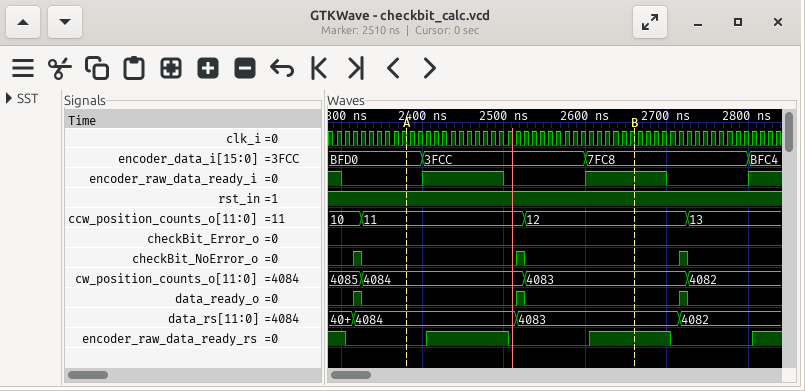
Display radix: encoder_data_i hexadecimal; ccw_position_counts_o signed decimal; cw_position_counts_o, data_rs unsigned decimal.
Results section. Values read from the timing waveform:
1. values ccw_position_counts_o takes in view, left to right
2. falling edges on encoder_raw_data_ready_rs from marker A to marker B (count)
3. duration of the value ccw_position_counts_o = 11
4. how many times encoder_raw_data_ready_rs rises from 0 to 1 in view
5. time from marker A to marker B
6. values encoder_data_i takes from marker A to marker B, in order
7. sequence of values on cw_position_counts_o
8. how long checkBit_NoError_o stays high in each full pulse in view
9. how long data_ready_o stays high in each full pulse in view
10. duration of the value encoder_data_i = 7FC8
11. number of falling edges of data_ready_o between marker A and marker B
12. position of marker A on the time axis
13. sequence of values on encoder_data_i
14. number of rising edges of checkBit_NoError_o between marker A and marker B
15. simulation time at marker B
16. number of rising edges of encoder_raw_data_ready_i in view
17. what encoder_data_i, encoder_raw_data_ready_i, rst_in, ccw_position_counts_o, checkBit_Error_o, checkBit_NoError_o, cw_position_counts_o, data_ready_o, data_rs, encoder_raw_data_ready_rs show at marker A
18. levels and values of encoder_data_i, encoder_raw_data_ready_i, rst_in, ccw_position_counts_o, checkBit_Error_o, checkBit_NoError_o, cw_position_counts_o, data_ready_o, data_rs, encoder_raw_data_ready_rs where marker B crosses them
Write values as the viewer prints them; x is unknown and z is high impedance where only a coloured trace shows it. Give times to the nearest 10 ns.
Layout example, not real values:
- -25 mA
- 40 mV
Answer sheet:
- 10, 11, 12, 13
- 1
- 200 ns
- 3
- 280 ns
- BFD0, 3FCC, 7FC8
- 4085, 4084, 4083, 4082
- 10 ns, 10 ns, 10 ns
- 10 ns, 10 ns, 10 ns
- 200 ns
- 1
- 2380 ns
- BFD0, 3FCC, 7FC8, BFC4
- 1
- 2660 ns
- 3
- encoder_data_i=BFD0, encoder_raw_data_ready_i=0, rst_in=1, ccw_position_counts_o=11, checkBit_Error_o=0, checkBit_NoError_o=0, cw_position_counts_o=4084, data_ready_o=0, data_rs=4084, encoder_raw_data_ready_rs=0
- encoder_data_i=7FC8, encoder_raw_data_ready_i=1, rst_in=1, ccw_position_counts_o=12, checkBit_Error_o=0, checkBit_NoError_o=0, cw_position_counts_o=4083, data_ready_o=0, data_rs=4083, encoder_raw_data_ready_rs=1
